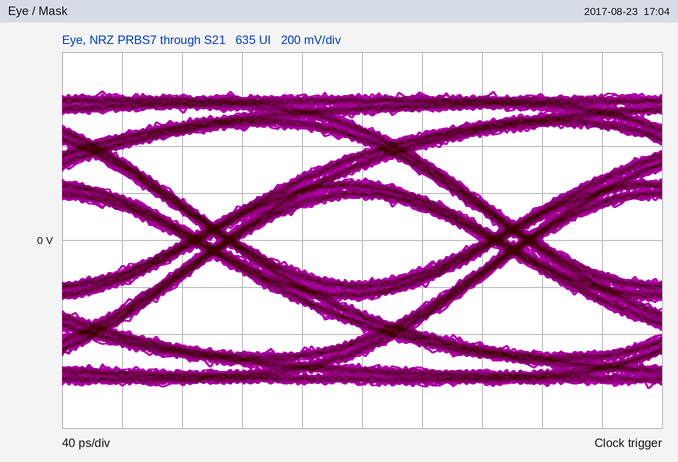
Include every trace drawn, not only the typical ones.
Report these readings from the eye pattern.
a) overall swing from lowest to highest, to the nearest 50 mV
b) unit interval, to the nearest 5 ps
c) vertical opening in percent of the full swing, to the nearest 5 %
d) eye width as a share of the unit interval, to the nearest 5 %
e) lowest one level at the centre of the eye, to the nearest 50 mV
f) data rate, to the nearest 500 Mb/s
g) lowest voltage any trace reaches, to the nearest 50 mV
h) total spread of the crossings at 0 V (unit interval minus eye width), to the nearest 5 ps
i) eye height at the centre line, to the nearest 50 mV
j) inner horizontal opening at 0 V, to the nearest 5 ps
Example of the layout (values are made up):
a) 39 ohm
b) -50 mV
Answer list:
a) 1.25 V
b) 200 ps
c) 30 %
d) 80 %
e) 200 mV
f) 5.0 Gb/s
g) -650 mV
h) 40 ps
i) 350 mV
j) 160 ps
